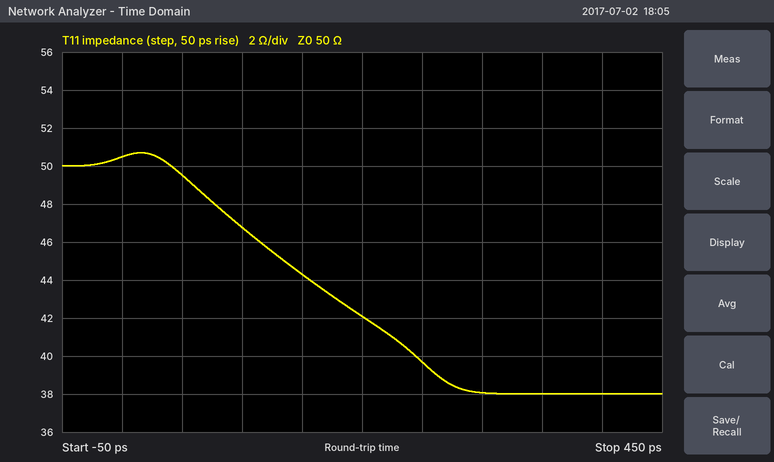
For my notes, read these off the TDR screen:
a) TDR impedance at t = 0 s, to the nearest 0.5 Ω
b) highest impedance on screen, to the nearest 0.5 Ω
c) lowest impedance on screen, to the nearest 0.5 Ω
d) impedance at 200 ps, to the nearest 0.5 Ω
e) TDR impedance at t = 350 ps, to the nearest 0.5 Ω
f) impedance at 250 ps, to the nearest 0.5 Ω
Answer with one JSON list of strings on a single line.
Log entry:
["50.5 Ω", "50.5 Ω", "38.0 Ω", "42.0 Ω", "38.0 Ω", "39.5 Ω"]
